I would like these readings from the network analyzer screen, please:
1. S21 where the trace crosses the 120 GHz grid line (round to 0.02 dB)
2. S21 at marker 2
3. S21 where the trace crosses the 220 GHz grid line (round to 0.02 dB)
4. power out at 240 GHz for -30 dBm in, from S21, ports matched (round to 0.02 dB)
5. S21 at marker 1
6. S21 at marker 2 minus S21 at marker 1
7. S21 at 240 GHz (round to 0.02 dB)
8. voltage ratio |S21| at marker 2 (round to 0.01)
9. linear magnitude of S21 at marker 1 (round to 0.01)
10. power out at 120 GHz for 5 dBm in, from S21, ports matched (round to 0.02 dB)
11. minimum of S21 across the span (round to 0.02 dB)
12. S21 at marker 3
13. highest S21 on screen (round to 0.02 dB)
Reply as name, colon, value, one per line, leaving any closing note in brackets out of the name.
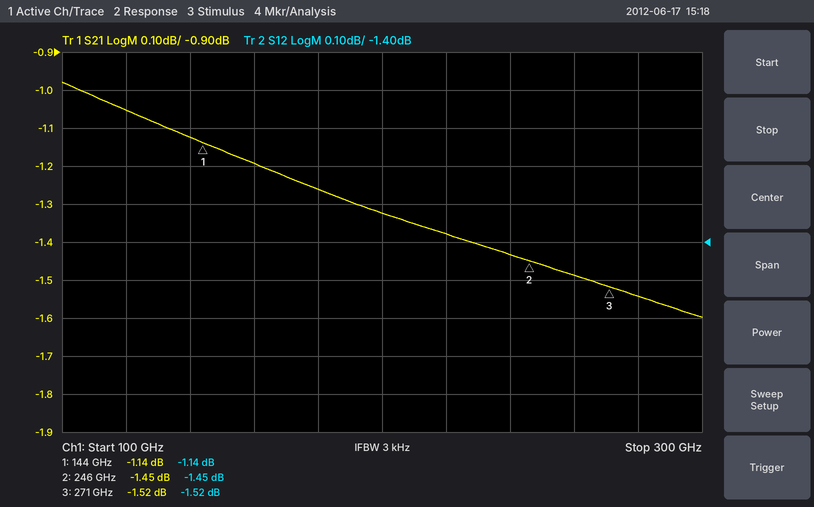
S21 where the trace crosses the 120 GHz grid line: -1.06 dB
S21 at marker 2: -1.45 dB
S21 where the trace crosses the 220 GHz grid line: -1.38 dB
power out at 240 GHz for -30 dBm in, from S21, ports matched: -31.44 dBm
S21 at marker 1: -1.14 dB
S21 at marker 2 minus S21 at marker 1: -0.31 dB
S21 at 240 GHz: -1.44 dB
voltage ratio |S21| at marker 2: 0.85
linear magnitude of S21 at marker 1: 0.88
power out at 120 GHz for 5 dBm in, from S21, ports matched: 3.94 dBm
minimum of S21 across the span: -1.60 dB
S21 at marker 3: -1.52 dB
highest S21 on screen: -0.98 dB
